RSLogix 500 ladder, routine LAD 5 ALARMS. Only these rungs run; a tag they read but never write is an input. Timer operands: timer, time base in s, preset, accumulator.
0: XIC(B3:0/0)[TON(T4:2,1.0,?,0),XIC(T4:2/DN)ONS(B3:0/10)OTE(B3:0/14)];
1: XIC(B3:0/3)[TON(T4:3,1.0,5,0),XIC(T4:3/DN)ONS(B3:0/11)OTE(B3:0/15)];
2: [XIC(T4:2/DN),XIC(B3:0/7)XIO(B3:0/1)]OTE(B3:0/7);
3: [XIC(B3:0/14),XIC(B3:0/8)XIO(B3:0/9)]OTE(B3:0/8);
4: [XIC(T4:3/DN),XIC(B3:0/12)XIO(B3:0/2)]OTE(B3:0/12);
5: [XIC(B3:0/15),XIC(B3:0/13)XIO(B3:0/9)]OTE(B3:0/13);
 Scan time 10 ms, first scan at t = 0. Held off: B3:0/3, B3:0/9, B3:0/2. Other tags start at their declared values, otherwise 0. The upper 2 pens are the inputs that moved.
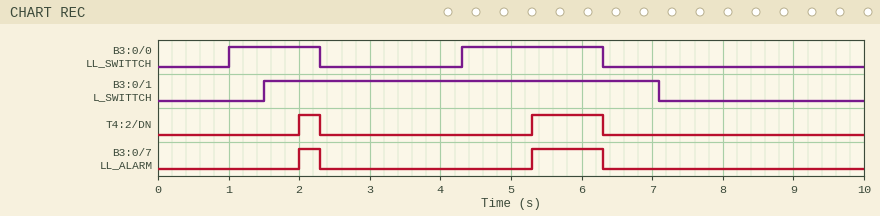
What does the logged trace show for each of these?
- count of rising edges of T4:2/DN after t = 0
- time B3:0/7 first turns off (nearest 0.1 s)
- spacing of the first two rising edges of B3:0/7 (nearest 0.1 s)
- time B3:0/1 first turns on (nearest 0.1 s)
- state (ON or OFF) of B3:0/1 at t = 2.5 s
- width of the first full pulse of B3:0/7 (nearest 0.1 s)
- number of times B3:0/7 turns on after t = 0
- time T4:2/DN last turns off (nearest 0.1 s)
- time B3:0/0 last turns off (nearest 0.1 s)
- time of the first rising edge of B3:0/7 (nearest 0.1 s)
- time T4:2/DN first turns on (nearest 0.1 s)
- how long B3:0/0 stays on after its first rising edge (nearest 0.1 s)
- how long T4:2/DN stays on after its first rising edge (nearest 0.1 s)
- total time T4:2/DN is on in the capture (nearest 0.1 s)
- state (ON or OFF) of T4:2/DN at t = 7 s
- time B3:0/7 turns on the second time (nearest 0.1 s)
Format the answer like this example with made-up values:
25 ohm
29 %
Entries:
2
2.3 s
3.3 s
1.5 s
ON
0.3 s
2
6.3 s
6.3 s
2.0 s
2.0 s
1.3 s
0.3 s
1.3 s
OFF
5.3 s
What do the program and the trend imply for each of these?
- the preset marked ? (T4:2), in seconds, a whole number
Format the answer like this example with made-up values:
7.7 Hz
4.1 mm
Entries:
1 s
